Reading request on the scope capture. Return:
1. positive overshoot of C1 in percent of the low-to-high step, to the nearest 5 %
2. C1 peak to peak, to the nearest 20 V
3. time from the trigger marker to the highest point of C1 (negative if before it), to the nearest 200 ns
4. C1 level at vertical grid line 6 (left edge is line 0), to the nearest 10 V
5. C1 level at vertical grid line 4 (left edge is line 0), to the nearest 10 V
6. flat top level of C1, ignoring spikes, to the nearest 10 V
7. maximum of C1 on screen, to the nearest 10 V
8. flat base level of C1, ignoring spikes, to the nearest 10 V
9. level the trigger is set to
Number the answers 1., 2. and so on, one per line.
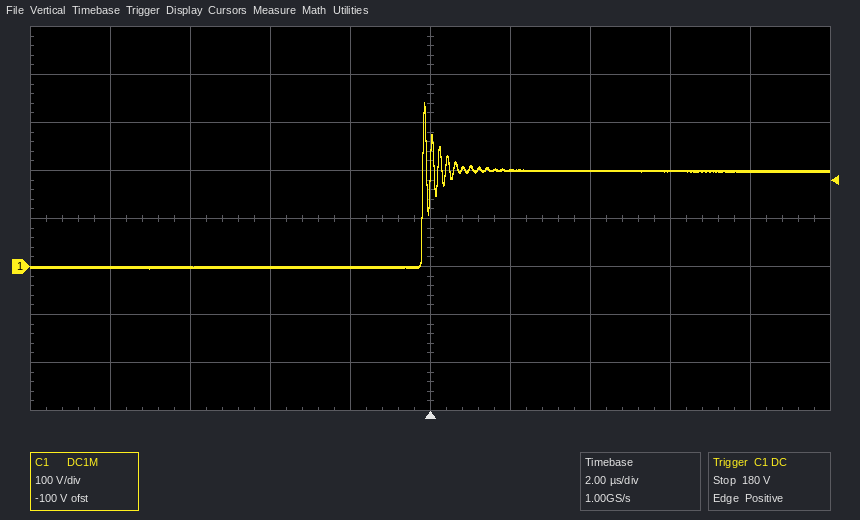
1. 70 %
2. 340 V
3. -200 ns
4. 200 V
5. 0 V
6. 200 V
7. 340 V
8. 0 V
9. 180 V
